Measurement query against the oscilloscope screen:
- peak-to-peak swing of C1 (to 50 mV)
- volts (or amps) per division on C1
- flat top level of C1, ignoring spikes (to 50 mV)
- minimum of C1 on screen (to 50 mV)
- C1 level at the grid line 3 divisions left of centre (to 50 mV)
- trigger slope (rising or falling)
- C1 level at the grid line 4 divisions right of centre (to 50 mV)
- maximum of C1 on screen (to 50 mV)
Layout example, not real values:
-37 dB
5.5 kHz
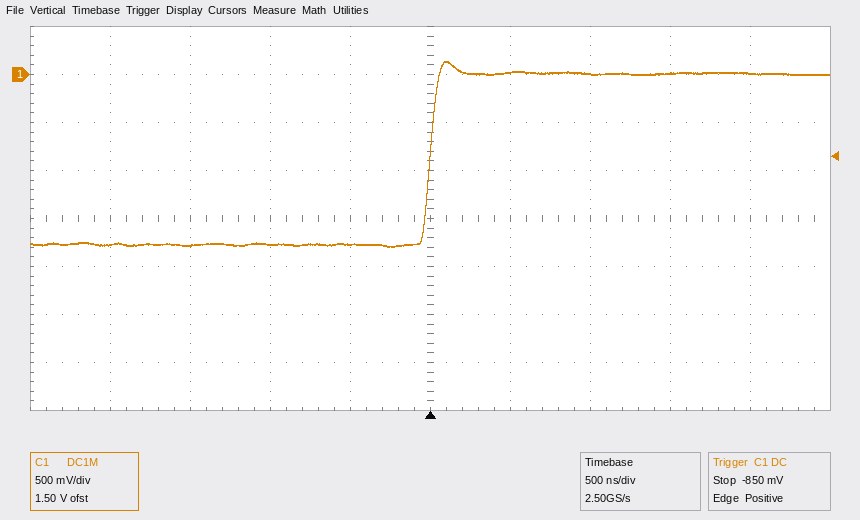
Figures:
1.95 V
500 mV
0 mV
-1.80 V
-1.80 V
rising
0 mV
150 mV
